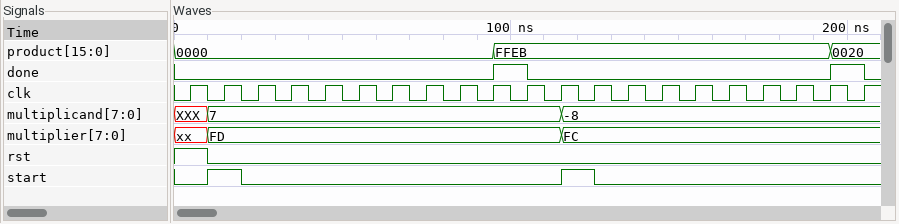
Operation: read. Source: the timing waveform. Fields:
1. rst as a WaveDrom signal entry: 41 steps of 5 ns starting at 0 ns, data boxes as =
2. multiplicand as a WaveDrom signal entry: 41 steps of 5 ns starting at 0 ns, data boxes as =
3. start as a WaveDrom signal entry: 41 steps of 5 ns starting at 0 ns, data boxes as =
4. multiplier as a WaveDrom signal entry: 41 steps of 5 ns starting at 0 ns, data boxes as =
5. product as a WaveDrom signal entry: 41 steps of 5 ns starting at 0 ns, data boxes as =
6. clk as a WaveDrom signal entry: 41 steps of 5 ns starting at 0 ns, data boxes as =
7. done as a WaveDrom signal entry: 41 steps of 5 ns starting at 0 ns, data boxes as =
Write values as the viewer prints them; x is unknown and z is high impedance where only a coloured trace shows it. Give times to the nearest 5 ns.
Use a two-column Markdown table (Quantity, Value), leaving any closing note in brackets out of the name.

| Quantity | Value |
|---|---|
| rst as a WaveDrom signal entry: 41 steps of 5 ns starting at 0 ns, data boxes as = | {name: 'rst', wave: '1.0......................................'} |
| multiplicand as a WaveDrom signal entry: 41 steps of 5 ns starting at 0 ns, data boxes as = | {name: 'multiplicand', wave: 'x.=....................=.................', data: '7 -8'} |
| start as a WaveDrom signal entry: 41 steps of 5 ns starting at 0 ns, data boxes as = | {name: 'start', wave: '0.1.0..................1.0...............'} |
| multiplier as a WaveDrom signal entry: 41 steps of 5 ns starting at 0 ns, data boxes as = | {name: 'multiplier', wave: 'x.=....................=.................', data: 'FD FC'} |
| product as a WaveDrom signal entry: 41 steps of 5 ns starting at 0 ns, data boxes as = | {name: 'product', wave: '=..................=...................=.', data: '0000 FFEB 0020'} |
| clk as a WaveDrom signal entry: 41 steps of 5 ns starting at 0 ns, data boxes as = | {name: 'clk', wave: '01010101010101010101010101010101010101010'} |
| done as a WaveDrom signal entry: 41 steps of 5 ns starting at 0 ns, data boxes as = | {name: 'done', wave: '0..................1.0.................1.'} |
